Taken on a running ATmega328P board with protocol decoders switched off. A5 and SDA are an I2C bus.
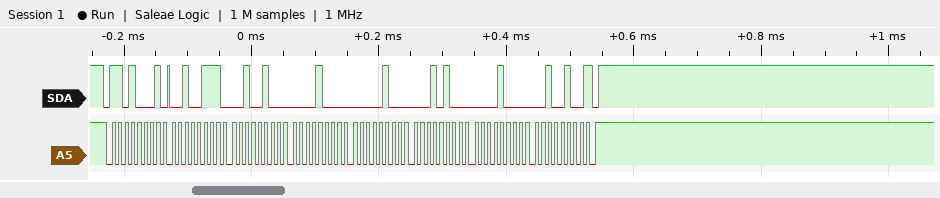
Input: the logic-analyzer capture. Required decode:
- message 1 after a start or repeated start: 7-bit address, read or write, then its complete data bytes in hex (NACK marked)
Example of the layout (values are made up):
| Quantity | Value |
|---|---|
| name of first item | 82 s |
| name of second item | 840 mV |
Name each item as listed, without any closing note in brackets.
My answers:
| Quantity | Value |
|---|---|
| message 1 after a start or repeated start: 7-bit address, read or write, then its complete data bytes in hex | 0x68 read: 27 24 08 04 14 08 24 NACK |
